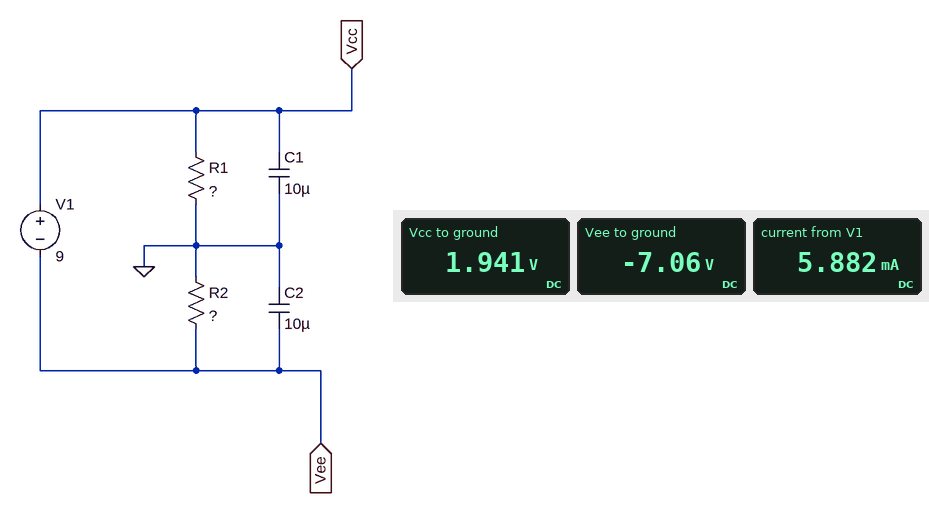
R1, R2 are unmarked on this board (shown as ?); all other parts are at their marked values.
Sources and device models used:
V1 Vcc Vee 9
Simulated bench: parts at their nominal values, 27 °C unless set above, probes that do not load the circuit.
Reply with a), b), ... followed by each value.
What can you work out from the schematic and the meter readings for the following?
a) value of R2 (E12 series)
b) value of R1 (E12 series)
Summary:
a) 1.2 kΩ
b) 330 Ω
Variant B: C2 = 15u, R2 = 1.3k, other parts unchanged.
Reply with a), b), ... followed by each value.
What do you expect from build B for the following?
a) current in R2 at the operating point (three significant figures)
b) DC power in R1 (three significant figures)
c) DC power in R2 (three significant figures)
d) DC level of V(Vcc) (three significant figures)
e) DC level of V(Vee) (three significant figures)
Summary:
a) 5.52 mA
b) 10.1 mW
c) 39.6 mW
d) 1.82 V
e) -7.18 V
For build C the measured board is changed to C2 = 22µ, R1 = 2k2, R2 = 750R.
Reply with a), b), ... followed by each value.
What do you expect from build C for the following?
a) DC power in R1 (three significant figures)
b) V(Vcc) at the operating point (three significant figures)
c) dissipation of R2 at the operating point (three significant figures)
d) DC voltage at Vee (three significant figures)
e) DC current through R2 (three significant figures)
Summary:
a) 20.5 mW
b) 6.71 V
c) 6.98 mW
d) -2.29 V
e) 3.05 mA
